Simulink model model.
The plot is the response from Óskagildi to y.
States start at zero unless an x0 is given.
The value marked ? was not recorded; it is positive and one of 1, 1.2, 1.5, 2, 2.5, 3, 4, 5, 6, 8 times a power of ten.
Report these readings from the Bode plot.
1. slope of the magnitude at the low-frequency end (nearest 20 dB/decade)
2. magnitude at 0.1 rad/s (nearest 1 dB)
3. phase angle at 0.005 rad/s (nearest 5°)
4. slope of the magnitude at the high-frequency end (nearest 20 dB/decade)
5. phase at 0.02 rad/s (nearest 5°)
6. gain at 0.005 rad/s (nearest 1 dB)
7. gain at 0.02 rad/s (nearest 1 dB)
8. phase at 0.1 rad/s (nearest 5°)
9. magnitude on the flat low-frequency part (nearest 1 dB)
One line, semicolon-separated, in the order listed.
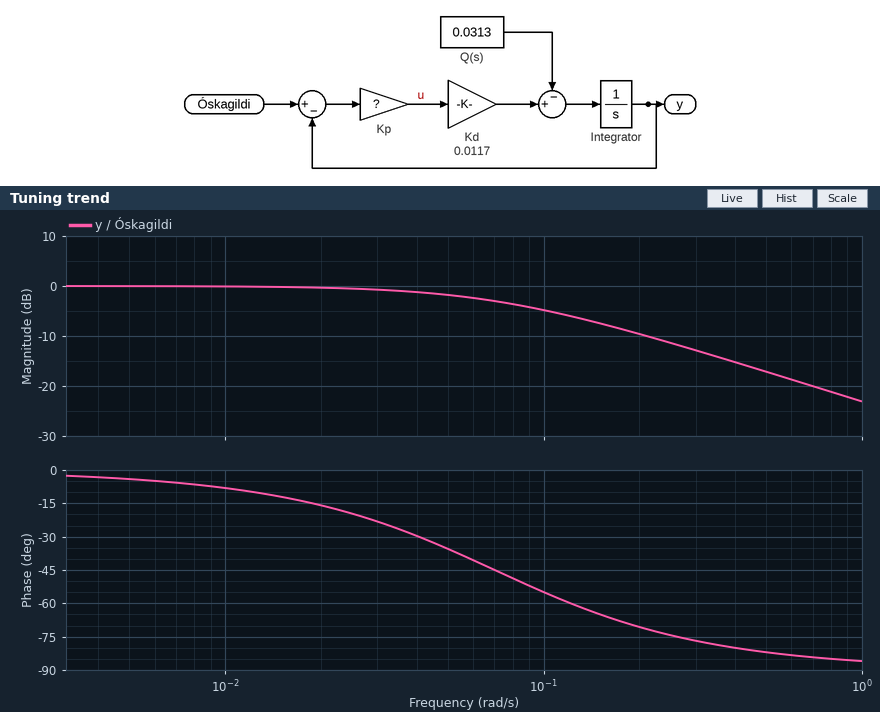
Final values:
0 dB/decade; -5 dB; -5°; -20 dB/decade; -15°; 0 dB; 0 dB; -55°; 0 dB
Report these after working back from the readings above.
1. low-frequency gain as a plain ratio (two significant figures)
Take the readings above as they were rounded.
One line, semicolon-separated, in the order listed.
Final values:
1.0
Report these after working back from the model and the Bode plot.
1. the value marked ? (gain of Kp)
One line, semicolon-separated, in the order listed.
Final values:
6
